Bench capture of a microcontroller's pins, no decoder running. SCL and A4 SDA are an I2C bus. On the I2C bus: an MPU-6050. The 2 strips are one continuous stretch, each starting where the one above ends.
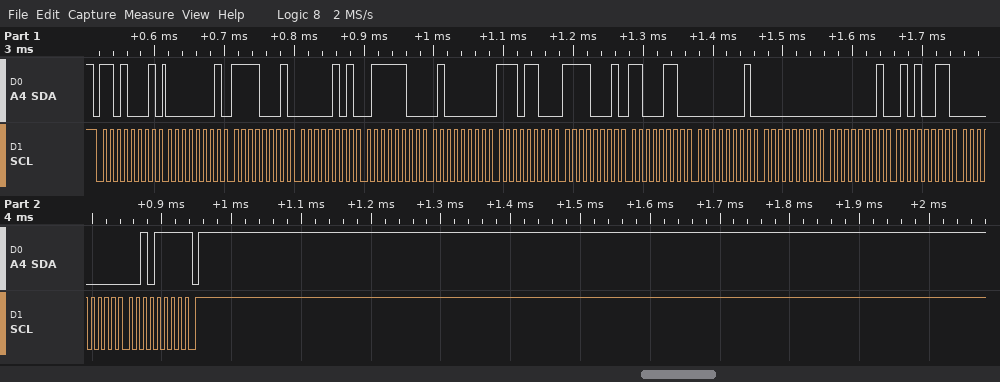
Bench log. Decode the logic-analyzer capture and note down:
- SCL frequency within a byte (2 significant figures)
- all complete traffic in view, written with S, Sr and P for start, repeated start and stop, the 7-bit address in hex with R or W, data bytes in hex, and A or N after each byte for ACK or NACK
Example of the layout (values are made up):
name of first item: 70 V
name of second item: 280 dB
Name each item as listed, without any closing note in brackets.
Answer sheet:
SCL frequency within a byte: 100 kHz
all complete traffic in view, written with S, Sr and P for start, repeated start and stop, the 7-bit address in hex with R or W, data bytes in hex, and A or N after each byte for ACK or NACK: S 68R A 01 A F1 A 05 A 7C A 40 A EC A F1 A C6 A 01 A 00 A 01 A 53 A 00 A 2F N P
